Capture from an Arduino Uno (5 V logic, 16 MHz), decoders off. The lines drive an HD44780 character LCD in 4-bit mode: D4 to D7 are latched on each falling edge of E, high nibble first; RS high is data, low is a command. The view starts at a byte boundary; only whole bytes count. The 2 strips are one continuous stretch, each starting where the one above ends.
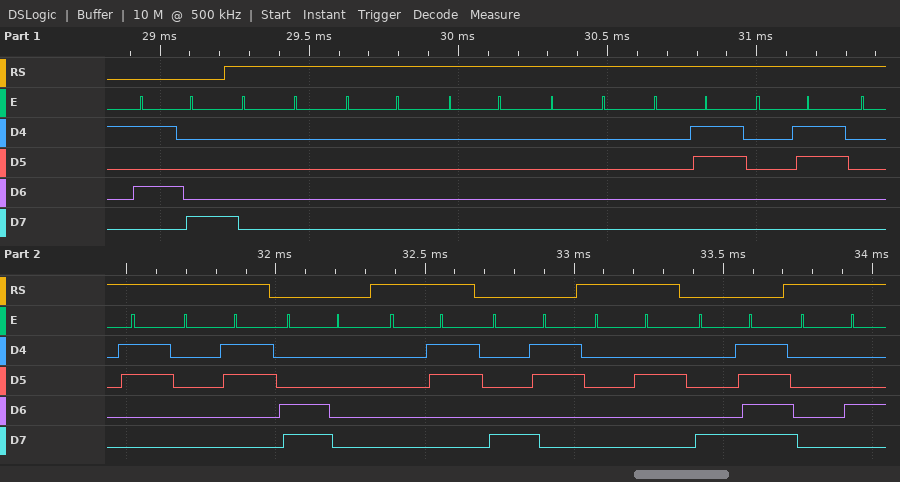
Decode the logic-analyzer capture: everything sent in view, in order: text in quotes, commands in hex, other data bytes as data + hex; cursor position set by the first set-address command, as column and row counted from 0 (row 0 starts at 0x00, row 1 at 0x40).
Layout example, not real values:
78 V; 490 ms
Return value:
0x58 data 00 00 00 00 03 03 03 03 0xC0 data 03 0x83 data 02 0x8F data 04; column 0, row 1
